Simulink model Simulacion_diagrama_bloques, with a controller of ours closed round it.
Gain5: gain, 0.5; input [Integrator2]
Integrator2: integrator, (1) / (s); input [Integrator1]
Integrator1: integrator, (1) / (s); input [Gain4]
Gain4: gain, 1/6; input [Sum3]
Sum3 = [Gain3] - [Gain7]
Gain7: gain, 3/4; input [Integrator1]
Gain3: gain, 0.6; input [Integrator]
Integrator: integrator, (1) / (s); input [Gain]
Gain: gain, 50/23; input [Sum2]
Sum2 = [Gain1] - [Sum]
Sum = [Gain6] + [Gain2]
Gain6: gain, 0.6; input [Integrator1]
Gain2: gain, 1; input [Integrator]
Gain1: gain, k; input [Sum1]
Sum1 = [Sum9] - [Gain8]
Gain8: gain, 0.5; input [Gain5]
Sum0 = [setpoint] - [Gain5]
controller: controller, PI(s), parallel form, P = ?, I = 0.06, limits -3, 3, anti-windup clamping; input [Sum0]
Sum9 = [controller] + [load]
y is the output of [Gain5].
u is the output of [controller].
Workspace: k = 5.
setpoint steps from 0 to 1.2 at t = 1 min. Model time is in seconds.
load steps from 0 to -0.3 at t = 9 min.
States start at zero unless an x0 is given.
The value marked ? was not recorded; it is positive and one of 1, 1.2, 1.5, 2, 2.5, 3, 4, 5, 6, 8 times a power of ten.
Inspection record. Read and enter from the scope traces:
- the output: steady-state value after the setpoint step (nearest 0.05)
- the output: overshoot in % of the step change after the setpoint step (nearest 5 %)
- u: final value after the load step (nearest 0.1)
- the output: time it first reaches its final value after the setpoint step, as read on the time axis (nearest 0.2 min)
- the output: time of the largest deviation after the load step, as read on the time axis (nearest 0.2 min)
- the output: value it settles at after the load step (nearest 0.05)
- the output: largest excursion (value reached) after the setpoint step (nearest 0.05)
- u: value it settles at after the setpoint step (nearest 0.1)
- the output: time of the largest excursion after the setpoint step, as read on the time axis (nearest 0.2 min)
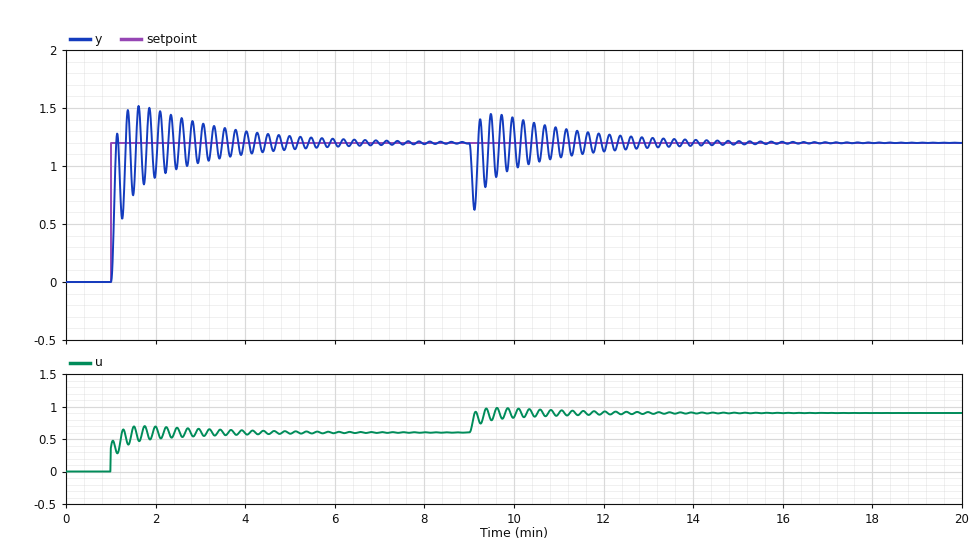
1.20
25 %
0.9
1.2 min
9.2 min
1.20
1.50
0.6
1.6 min
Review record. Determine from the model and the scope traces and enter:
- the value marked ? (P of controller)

0.3
